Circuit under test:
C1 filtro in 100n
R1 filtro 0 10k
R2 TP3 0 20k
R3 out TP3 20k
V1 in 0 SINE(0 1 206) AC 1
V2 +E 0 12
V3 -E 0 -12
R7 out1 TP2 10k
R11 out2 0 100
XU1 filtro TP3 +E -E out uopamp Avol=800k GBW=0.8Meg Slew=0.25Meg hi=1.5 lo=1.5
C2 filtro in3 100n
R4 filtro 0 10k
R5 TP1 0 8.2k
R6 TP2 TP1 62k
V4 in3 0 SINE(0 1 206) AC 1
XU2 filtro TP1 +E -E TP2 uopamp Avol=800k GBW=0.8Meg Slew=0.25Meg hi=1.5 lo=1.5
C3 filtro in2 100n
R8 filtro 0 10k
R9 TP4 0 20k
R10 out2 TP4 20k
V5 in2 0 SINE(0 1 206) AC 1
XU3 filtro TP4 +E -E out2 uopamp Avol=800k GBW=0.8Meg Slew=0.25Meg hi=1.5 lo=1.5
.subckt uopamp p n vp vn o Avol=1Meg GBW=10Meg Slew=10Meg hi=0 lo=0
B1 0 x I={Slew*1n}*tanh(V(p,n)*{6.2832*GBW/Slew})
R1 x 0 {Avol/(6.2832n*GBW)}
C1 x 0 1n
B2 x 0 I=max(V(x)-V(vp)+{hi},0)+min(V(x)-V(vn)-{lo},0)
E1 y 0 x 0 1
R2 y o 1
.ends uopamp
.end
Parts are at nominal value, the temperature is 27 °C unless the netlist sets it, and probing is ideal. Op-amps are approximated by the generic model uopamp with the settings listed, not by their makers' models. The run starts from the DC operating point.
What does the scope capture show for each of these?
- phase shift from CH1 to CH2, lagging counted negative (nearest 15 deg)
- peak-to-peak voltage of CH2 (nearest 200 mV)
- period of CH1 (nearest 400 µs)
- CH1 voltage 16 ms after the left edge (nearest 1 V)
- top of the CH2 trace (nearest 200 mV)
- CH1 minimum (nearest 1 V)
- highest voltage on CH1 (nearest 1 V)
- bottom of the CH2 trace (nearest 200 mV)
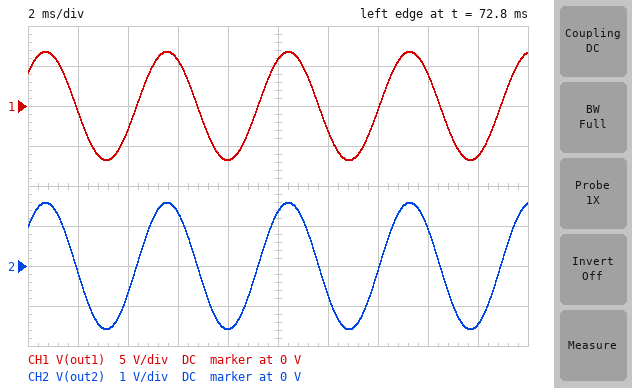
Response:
0 deg
3.2 V
4.8 ms
4 V
1.6 V
-7 V
7 V
-1.6 V
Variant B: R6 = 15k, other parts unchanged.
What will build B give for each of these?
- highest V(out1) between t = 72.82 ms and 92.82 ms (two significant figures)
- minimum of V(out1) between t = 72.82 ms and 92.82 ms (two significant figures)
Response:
2.2 V
-2.2 V
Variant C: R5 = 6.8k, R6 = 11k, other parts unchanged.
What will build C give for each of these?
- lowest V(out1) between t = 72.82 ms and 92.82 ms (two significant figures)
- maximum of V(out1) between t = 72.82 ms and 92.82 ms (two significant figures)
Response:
-2.1 V
2.1 V
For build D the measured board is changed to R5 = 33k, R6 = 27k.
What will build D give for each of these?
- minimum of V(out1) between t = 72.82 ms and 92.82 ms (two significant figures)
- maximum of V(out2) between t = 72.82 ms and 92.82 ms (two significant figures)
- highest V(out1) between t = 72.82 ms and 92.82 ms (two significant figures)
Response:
-1.4 V
1.6 V
1.4 V
